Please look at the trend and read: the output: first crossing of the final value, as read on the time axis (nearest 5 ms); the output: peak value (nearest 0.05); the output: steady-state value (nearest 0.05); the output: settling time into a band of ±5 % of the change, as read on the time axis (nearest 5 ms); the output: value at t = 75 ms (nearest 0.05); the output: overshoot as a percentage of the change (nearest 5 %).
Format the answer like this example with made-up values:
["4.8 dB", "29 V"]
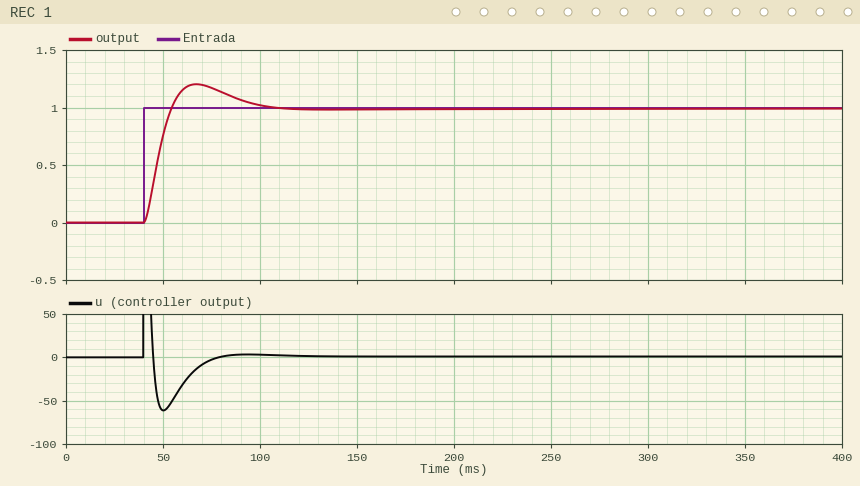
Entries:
["55 ms", "1.20", "1.00", "95 ms", "1.15", "20 %"]
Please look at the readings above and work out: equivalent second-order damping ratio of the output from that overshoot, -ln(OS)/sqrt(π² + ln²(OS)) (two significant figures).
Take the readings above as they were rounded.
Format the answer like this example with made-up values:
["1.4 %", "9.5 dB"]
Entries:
["0.46"]
